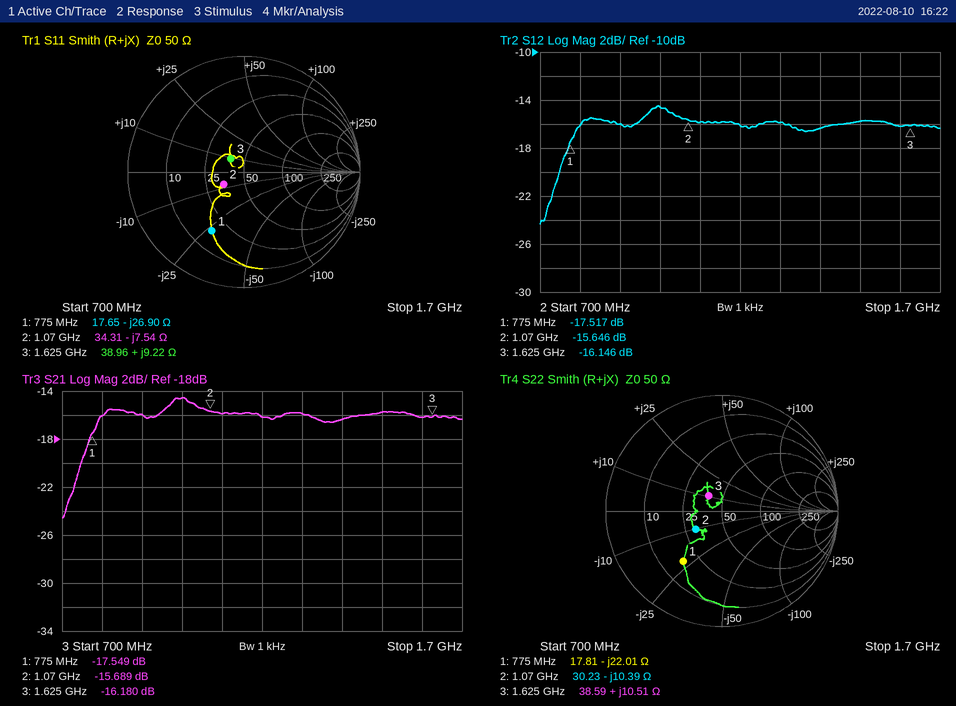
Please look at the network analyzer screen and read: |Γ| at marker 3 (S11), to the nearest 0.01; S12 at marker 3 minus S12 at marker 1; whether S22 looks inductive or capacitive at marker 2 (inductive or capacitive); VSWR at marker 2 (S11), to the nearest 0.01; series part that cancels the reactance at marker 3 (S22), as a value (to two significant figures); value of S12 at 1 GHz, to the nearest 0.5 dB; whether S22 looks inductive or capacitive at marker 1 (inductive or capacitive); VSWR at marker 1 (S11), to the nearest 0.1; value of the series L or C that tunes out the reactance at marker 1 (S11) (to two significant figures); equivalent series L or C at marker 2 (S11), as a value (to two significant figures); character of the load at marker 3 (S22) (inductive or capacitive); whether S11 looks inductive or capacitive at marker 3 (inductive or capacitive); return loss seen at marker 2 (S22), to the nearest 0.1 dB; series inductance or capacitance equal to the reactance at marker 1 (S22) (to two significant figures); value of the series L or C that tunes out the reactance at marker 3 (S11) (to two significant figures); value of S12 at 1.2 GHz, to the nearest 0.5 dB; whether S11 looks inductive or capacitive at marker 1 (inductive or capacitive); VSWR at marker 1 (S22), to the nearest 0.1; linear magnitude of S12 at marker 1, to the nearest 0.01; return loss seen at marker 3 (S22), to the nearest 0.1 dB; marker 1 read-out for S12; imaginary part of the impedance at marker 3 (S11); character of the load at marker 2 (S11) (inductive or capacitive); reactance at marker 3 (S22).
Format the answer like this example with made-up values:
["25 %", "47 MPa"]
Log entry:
["0.16", "1.371 dB", "capacitive", "1.52", "9.3 pF", "-14.5 dB", "capacitive", "3.7", "5.5 nH", "20 pF", "inductive", "inductive", "11.2 dB", "9.3 pF", "11 pF", "-16.0 dB", "capacitive", "3.4", "0.13", "15.2 dB", "-17.517 dB", "+9.22 Ω", "capacitive", "+10.51 Ω"]
